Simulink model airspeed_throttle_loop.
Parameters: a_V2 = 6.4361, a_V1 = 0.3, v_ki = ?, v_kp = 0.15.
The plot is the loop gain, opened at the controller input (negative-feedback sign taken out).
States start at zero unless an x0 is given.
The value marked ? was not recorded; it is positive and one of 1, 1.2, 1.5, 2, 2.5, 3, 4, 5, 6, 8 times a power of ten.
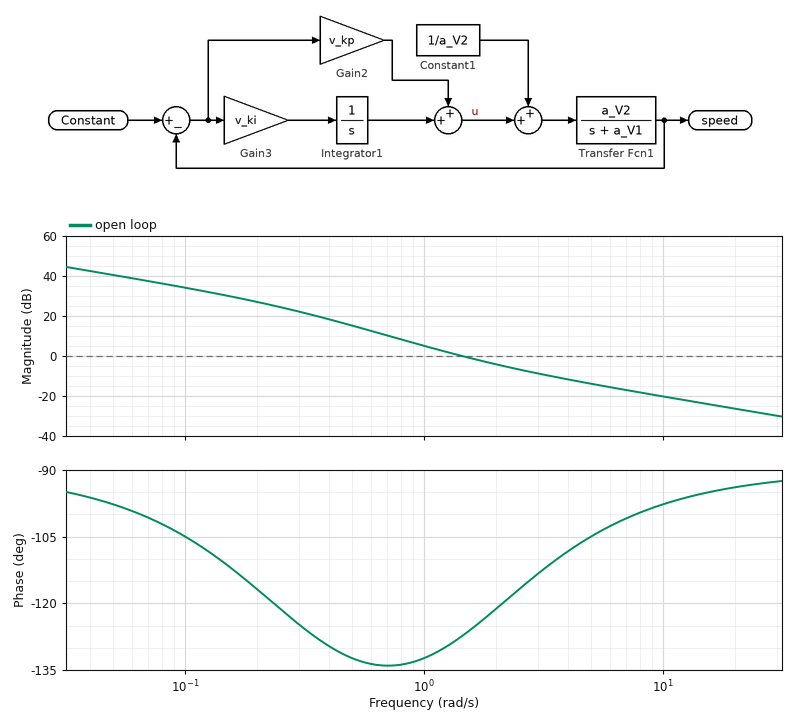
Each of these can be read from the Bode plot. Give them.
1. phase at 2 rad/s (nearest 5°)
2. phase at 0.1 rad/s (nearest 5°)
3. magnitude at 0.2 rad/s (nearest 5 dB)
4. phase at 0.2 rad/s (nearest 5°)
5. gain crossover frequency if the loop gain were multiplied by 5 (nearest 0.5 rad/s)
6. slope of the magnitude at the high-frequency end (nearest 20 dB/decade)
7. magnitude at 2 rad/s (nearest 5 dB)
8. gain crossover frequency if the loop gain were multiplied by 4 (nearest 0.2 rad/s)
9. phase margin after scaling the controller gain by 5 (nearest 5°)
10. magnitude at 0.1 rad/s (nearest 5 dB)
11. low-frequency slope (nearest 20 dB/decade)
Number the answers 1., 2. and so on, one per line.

1. -120°
2. -105°
3. 25 dB
4. -115°
5. 5.0 rad/s
6. -20 dB/decade
7. -5 dB
8. 4.2 rad/s
9. 75°
10. 35 dB
11. -20 dB/decade
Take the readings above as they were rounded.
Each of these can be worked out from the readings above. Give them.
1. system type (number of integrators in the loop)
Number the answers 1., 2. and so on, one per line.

1. 1
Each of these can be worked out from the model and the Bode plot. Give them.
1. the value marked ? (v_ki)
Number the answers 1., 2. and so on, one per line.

1. 0.25
